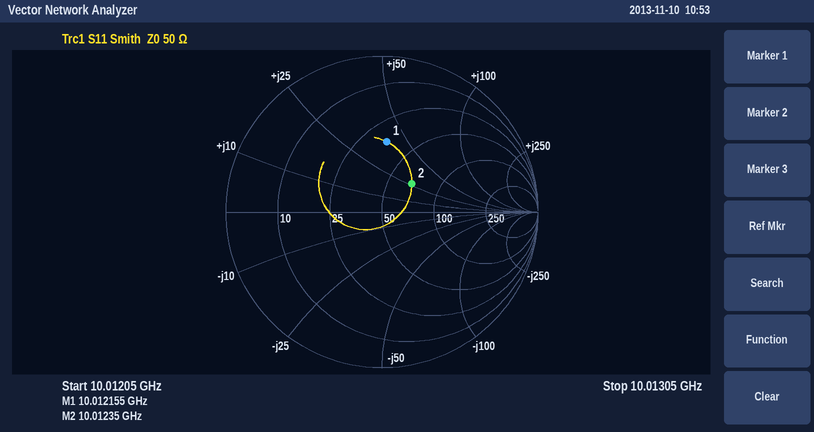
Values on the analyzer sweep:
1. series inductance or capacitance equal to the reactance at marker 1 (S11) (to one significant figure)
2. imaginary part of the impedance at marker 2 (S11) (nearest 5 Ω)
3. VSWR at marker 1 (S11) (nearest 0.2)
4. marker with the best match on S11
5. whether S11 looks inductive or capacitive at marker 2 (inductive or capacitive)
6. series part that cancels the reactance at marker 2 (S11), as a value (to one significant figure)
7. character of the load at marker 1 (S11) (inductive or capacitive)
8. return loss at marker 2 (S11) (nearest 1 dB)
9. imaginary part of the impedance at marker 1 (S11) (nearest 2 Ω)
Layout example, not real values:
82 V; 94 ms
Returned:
600 pH; +25 Ω; 2.6; marker 2; inductive; 600 fF; inductive; 12 dB; +40 Ω
